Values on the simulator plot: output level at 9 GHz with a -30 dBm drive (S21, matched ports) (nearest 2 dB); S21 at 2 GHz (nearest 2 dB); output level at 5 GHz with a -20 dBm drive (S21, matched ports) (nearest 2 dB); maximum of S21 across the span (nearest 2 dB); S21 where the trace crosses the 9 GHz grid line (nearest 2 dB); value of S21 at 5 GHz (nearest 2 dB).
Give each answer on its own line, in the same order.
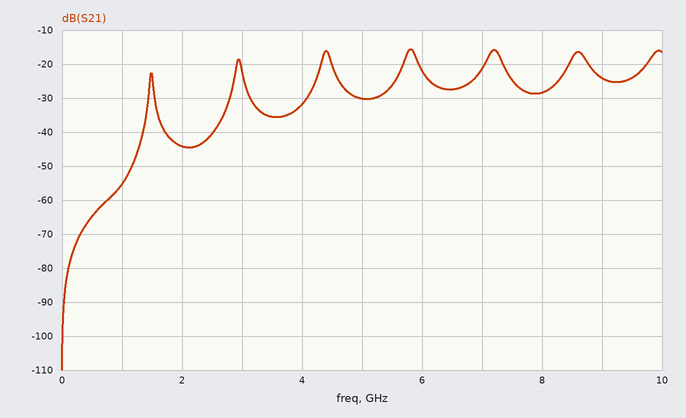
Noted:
-54 dBm
-44 dB
-50 dBm
-16 dB
-24 dB
-30 dB
